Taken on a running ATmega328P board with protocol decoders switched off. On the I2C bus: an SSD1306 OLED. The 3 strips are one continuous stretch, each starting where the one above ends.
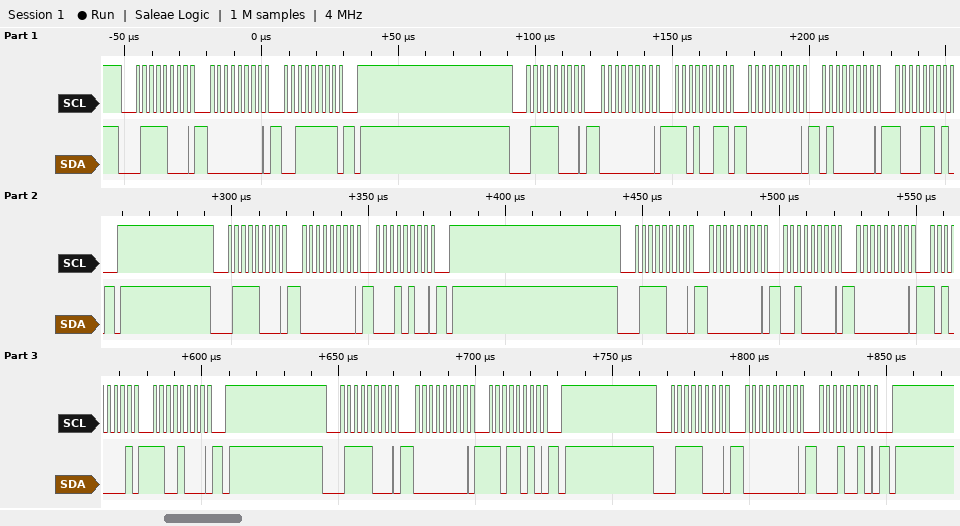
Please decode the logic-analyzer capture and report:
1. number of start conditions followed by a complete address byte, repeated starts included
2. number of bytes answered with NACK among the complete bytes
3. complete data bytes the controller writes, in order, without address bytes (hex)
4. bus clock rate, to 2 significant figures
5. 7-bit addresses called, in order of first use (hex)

6
0
00 3F 00 D3 00 40 8D 00 14 00 20 00 A1 C8 00 DA 00 12
400 kHz
0x3C
